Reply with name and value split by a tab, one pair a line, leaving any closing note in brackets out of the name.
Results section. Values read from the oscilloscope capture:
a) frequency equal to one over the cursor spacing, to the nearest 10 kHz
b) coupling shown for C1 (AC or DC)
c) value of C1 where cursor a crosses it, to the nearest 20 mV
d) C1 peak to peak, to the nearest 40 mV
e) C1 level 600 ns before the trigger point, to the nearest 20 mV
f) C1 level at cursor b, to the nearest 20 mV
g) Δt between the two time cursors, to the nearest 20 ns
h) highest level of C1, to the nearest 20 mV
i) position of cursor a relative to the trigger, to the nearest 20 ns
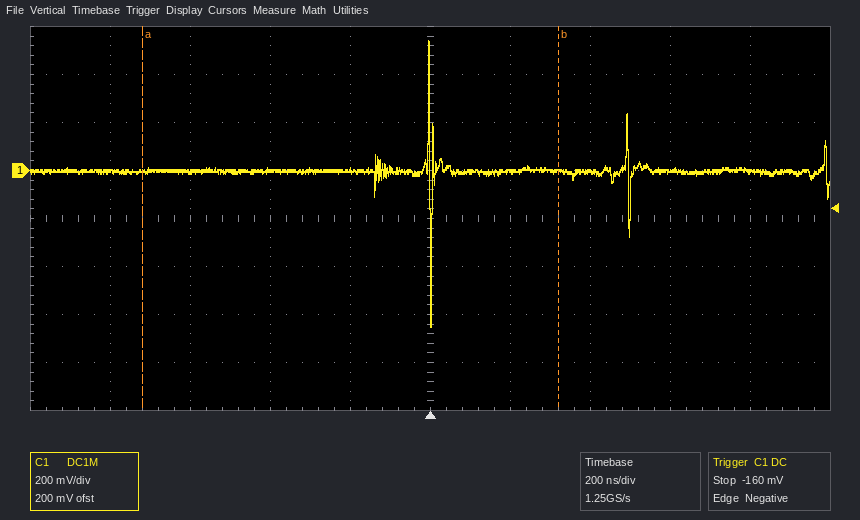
frequency equal to one over the cursor spacing, to the nearest 10 kHz	960 kHz
coupling shown for C1	DC
value of C1 where cursor a crosses it, to the nearest 20 mV	0 mV
C1 peak to peak, to the nearest 40 mV	1.20 V
C1 level 600 ns before the trigger point, to the nearest 20 mV	0 mV
C1 level at cursor b, to the nearest 20 mV	0 mV
Δt between the two time cursors, to the nearest 20 ns	1.04 µs
highest level of C1, to the nearest 20 mV	540 mV
position of cursor a relative to the trigger, to the nearest 20 ns	-720 ns
